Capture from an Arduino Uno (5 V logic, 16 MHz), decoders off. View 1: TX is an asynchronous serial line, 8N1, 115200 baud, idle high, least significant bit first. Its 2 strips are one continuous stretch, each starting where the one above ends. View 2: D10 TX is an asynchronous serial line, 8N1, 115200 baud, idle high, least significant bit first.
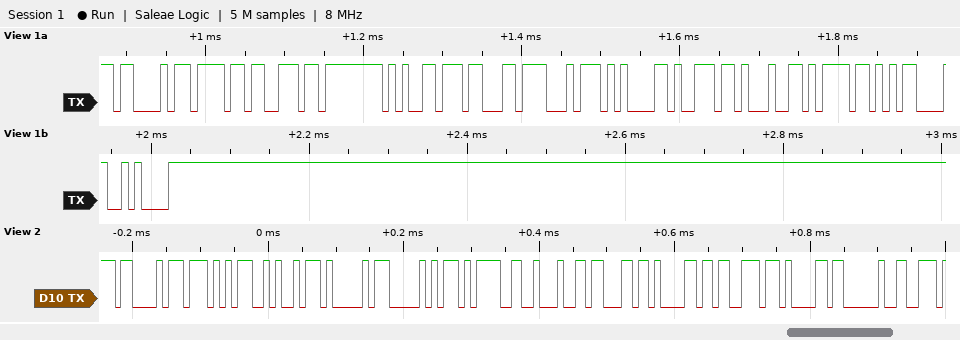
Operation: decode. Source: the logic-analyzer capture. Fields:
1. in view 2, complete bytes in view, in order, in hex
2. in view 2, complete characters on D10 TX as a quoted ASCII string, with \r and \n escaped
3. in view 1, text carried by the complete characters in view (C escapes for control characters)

43 57 4A 41 50 3D 22 63 61 73 61 20
"CWJAP=\"casa "
"Conectando\r\n"
